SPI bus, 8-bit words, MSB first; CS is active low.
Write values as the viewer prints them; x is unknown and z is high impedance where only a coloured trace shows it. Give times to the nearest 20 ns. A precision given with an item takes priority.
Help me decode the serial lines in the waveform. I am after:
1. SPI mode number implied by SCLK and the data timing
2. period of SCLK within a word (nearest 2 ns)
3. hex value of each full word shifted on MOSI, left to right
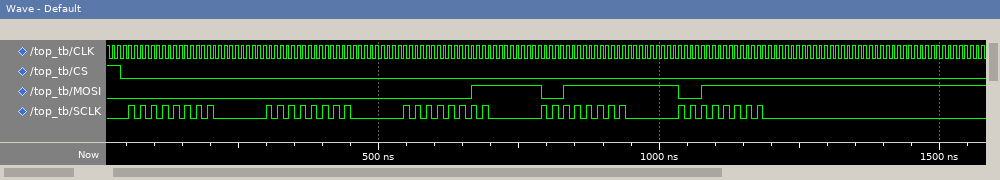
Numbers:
1
20 ns
00, 00, 03, 3F, 3F
